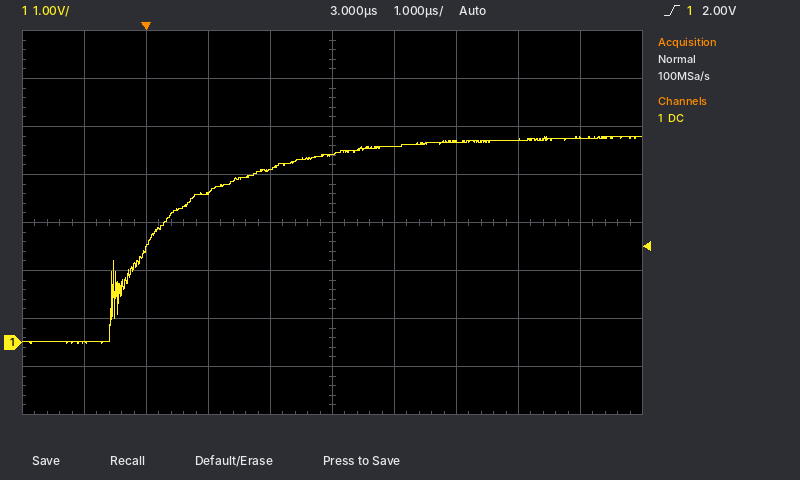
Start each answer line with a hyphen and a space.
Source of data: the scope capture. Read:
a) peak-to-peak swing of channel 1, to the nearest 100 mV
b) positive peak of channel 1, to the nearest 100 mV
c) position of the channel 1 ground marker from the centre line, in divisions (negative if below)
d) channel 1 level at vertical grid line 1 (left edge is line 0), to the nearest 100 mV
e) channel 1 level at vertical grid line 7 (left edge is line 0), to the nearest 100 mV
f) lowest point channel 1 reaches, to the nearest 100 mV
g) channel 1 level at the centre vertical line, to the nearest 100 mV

- 4.3 V
- 4.3 V
- -2.5 div
- 0.0 V
- 4.2 V
- 0.0 V
- 3.9 V
